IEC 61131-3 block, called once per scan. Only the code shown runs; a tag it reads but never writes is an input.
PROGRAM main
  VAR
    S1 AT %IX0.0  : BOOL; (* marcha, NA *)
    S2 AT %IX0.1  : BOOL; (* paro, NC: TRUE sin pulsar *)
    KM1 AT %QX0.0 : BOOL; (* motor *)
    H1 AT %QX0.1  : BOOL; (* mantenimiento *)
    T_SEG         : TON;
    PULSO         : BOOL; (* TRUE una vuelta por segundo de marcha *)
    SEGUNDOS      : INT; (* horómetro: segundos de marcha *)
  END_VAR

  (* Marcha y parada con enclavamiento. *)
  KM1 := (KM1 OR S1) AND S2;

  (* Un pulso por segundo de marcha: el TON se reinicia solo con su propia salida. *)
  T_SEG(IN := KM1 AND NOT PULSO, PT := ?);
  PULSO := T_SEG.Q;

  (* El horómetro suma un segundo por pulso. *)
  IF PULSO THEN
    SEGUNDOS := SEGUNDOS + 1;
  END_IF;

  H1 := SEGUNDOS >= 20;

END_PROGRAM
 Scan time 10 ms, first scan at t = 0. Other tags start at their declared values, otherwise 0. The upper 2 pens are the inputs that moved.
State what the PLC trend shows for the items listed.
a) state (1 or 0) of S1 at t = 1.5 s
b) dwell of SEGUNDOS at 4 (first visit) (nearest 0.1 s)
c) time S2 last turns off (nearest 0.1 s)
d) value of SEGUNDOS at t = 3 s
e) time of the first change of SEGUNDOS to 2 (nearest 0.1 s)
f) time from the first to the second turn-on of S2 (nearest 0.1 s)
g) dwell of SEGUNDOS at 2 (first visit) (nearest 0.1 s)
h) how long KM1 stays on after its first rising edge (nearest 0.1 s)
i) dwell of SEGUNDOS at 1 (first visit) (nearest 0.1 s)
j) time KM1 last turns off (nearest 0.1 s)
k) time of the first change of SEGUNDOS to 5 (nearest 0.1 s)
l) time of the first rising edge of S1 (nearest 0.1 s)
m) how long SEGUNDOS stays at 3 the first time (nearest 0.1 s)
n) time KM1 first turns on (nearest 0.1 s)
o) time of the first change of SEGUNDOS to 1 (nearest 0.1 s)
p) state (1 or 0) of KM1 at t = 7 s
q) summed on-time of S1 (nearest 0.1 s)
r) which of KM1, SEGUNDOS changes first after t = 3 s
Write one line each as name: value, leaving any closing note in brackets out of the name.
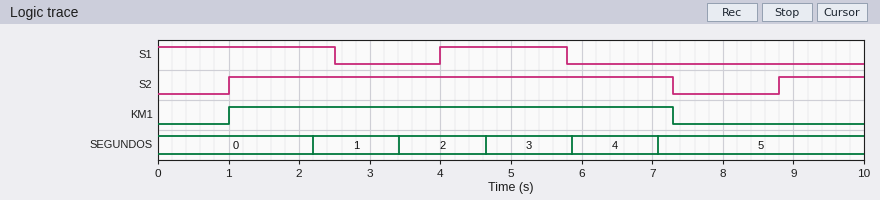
state (1 or 0) of S1 at t = 1.5 s: 1
dwell of SEGUNDOS at 4 (first visit): 1.2 s
time S2 last turns off: 7.3 s
value of SEGUNDOS at t = 3 s: 1
time of the first change of SEGUNDOS to 2: 3.4 s
time from the first to the second turn-on of S2: 7.8 s
dwell of SEGUNDOS at 2 (first visit): 1.2 s
how long KM1 stays on after its first rising edge: 6.3 s
dwell of SEGUNDOS at 1 (first visit): 1.2 s
time KM1 last turns off: 7.3 s
time of the first change of SEGUNDOS to 5: 7.1 s
time of the first rising edge of S1: 4.0 s
how long SEGUNDOS stays at 3 the first time: 1.2 s
time KM1 first turns on: 1.0 s
time of the first change of SEGUNDOS to 1: 2.2 s
state (1 or 0) of KM1 at t = 7 s: 1
summed on-time of S1: 4.3 s
which of KM1, SEGUNDOS changes first after t = 3 s: SEGUNDOS
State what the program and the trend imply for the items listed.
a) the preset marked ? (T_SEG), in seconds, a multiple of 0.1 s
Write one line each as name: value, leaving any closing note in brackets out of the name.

the preset marked ? (T_SEG), in seconds, a multiple of 0.1 s: 1.2 s
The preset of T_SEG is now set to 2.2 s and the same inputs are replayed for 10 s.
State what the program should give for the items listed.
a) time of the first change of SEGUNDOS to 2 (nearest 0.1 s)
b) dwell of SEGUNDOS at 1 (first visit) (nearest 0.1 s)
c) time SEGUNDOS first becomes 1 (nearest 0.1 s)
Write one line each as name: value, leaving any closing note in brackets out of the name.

time of the first change of SEGUNDOS to 2: 5.4 s
dwell of SEGUNDOS at 1 (first visit): 2.2 s
time SEGUNDOS first becomes 1: 3.2 s
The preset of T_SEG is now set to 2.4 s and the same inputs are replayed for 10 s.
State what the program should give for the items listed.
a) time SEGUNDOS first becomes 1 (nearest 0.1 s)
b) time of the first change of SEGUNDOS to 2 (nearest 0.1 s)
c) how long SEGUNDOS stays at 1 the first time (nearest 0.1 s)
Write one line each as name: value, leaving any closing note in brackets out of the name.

time SEGUNDOS first becomes 1: 3.4 s
time of the first change of SEGUNDOS to 2: 5.8 s
how long SEGUNDOS stays at 1 the first time: 2.4 s
